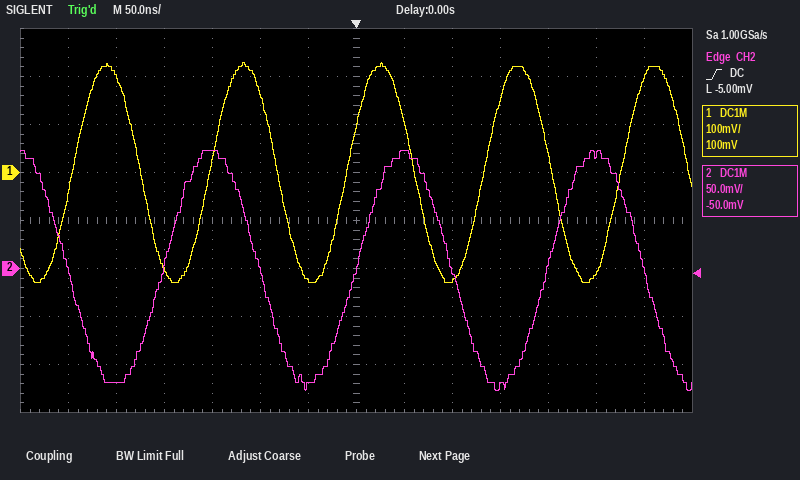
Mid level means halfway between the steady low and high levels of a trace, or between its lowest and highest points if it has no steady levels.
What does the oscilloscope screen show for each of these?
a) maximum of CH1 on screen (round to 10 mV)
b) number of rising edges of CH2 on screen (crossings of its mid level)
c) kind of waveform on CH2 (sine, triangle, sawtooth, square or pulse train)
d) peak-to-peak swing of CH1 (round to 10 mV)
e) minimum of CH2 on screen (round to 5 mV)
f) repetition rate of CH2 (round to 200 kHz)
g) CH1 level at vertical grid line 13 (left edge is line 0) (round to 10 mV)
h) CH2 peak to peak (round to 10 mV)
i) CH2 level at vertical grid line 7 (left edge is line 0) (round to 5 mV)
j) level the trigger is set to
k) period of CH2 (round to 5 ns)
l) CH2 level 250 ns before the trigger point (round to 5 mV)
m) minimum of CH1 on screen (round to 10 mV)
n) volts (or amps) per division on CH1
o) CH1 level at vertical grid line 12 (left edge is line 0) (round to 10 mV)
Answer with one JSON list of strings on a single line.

["230 mV", "3", "sine", "460 mV", "-125 mV", "5.0 MHz", "200 mV", "250 mV", "0 mV", "-5.00 mV", "200 ns", "-120 mV", "-230 mV", "100 mV", "-210 mV"]
